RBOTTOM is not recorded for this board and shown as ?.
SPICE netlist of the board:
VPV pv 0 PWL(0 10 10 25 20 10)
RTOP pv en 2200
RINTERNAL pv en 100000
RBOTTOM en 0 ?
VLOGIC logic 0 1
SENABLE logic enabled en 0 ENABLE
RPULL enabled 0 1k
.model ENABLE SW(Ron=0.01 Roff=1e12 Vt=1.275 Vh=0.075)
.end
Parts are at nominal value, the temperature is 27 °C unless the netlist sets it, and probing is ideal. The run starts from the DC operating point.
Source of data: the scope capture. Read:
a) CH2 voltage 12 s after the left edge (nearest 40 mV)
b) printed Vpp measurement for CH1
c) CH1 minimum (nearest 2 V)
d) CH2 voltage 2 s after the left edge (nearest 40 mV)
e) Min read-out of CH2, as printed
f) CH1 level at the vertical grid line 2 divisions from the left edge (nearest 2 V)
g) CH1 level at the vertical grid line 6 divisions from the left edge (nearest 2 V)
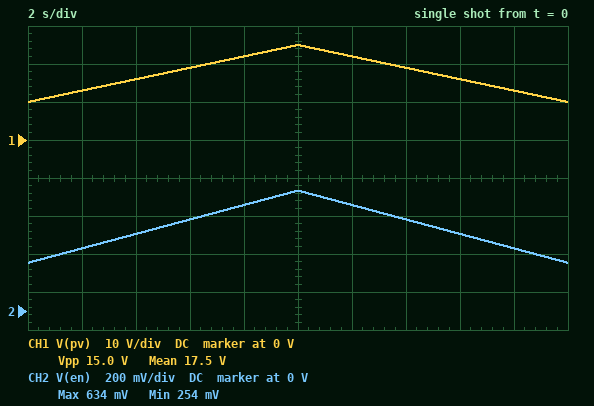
560 mV
15.0 V
10 V
320 mV
254 mV
16 V
22 V
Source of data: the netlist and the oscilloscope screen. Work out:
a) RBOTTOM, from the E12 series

56 Ω
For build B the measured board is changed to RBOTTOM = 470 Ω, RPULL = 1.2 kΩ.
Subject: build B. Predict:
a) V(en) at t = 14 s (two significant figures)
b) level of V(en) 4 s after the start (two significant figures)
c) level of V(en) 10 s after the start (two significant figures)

3.4 V
2.9 V
4.5 V
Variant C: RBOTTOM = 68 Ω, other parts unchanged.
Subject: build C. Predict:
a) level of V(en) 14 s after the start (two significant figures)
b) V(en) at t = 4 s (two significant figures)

580 mV
490 mV
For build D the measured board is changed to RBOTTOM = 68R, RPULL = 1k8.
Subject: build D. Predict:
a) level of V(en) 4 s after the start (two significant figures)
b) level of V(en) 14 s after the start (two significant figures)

490 mV
580 mV
